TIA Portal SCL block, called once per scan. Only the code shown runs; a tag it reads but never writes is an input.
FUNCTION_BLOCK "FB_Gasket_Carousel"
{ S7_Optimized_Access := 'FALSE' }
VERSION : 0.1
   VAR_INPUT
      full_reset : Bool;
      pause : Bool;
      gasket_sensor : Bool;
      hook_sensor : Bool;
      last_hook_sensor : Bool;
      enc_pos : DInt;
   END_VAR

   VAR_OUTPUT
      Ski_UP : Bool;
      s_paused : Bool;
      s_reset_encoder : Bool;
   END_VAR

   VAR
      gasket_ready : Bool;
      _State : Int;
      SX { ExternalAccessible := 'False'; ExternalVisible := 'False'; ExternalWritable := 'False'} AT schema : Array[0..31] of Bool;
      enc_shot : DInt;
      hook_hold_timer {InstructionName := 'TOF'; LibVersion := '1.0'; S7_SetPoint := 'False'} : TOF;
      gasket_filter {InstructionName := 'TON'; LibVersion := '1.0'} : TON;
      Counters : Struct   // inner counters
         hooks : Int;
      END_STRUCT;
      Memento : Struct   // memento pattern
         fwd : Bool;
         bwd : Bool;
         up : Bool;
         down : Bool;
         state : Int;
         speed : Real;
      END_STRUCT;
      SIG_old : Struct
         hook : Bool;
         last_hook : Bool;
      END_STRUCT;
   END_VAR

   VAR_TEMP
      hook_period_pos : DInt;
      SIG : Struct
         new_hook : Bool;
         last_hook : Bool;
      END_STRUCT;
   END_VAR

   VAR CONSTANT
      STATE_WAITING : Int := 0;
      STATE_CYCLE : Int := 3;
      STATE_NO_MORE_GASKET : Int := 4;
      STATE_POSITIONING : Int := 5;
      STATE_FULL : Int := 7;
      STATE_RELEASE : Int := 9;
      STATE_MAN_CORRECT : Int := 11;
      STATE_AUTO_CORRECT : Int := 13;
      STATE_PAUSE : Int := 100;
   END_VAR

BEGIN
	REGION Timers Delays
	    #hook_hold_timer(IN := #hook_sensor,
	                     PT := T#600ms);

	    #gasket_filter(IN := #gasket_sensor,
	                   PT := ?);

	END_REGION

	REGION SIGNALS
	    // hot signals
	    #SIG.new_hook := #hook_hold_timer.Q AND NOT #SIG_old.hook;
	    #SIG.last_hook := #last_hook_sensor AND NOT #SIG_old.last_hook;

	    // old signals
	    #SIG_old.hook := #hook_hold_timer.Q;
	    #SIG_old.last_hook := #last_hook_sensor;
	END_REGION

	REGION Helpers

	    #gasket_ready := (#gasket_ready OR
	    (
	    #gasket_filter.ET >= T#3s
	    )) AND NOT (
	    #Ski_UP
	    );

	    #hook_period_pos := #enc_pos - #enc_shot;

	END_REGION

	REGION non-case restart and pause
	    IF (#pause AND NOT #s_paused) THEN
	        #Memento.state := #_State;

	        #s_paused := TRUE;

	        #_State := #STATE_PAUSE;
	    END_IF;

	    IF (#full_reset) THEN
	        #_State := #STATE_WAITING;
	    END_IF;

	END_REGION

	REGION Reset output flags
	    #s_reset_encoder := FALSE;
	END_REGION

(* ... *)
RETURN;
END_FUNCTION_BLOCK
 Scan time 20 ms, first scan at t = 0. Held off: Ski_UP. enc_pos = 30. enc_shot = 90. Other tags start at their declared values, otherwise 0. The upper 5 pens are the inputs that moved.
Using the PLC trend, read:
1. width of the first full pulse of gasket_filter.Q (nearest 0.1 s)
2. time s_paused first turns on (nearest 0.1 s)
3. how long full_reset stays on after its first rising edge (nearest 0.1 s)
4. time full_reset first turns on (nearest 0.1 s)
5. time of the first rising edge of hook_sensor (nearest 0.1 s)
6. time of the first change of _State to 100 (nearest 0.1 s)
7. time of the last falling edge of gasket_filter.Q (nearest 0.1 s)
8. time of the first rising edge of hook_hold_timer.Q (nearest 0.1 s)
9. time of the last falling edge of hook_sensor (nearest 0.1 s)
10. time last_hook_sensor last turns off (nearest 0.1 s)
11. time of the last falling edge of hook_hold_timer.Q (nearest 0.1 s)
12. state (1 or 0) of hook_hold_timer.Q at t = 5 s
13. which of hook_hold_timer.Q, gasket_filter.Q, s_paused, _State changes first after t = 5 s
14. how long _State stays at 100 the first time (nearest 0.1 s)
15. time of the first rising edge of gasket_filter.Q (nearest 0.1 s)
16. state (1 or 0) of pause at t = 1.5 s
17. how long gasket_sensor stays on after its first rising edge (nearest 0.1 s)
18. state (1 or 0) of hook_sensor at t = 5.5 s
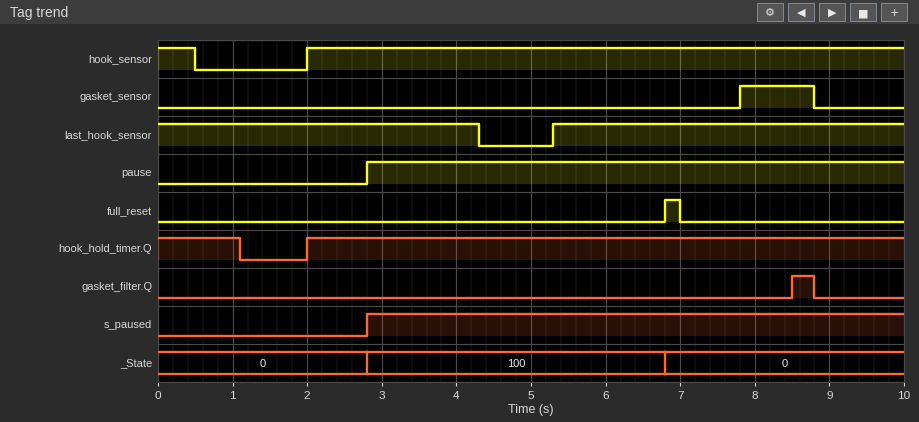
0.3 s
2.8 s
0.2 s
6.8 s
2.0 s
2.8 s
8.8 s
2.0 s
0.5 s
4.3 s
1.1 s
1
_State
4.0 s
8.5 s
0
1.0 s
1
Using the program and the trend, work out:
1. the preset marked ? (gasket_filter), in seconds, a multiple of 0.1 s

0.7 s
